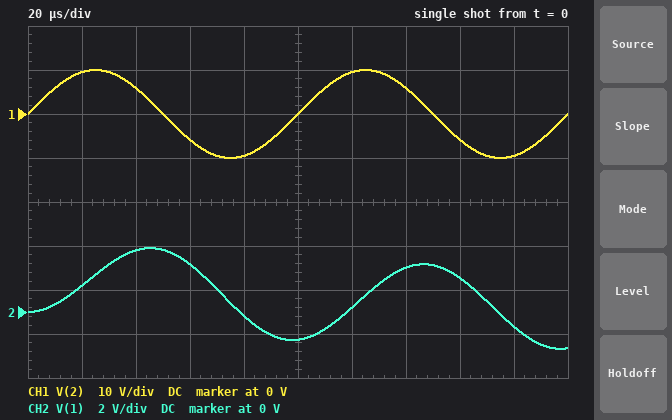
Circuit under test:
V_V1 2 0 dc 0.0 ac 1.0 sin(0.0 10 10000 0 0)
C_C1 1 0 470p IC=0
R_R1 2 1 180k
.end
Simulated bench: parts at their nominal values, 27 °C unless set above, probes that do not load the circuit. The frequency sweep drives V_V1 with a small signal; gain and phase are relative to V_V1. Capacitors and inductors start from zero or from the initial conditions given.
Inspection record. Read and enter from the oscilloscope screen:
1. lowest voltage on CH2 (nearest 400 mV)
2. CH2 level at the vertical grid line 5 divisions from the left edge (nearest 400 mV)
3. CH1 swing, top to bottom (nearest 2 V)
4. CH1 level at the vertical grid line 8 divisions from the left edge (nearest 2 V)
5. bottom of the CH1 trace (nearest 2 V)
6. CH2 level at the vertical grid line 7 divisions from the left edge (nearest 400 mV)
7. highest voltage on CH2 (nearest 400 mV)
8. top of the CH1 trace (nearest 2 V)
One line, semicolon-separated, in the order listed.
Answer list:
-1.6 V; -1.2 V; 20 V; -6 V; -10 V; 2.0 V; 2.8 V; 10 V
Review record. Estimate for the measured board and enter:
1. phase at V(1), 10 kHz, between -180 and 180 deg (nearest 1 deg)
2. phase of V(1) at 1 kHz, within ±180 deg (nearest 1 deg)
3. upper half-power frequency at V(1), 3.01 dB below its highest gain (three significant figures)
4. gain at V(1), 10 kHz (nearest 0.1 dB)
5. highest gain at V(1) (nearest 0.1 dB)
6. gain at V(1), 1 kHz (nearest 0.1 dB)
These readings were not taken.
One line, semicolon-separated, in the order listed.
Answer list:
-79 deg; -28 deg; 1.88 kHz; -14.7 dB; 0 dB; -1.1 dB
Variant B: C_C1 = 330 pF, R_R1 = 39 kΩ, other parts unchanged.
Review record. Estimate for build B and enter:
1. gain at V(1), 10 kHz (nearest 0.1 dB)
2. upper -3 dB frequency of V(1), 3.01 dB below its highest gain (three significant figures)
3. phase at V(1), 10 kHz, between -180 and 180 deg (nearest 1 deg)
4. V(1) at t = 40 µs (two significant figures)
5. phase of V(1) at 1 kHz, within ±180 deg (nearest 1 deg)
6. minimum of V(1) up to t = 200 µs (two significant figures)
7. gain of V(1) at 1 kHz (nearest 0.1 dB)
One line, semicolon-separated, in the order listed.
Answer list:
-2.2 dB; 12.4 kHz; -39 deg; 7.7 V; -5 deg; -7.8 V; 0 dB
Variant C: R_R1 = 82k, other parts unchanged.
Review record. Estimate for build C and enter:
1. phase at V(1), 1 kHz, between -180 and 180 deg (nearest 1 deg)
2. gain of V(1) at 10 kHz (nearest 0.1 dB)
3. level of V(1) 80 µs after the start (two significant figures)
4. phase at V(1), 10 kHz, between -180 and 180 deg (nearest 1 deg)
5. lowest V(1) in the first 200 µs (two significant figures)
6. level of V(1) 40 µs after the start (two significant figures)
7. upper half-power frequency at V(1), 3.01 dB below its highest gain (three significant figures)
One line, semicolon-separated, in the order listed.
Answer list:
-14 deg; -8.4 dB; -2.0 V; -68 deg; -3.8 V; 5.0 V; 4.13 kHz
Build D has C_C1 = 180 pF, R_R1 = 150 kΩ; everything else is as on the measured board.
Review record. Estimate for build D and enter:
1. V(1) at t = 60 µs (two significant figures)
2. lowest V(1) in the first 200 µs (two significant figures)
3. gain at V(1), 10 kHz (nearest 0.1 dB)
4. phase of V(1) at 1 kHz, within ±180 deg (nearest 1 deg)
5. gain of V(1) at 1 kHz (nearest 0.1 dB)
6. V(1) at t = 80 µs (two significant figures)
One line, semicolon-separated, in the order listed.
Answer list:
2.5 V; -5.1 V; -5.9 dB; -10 deg; -0.1 dB; -3.6 V
